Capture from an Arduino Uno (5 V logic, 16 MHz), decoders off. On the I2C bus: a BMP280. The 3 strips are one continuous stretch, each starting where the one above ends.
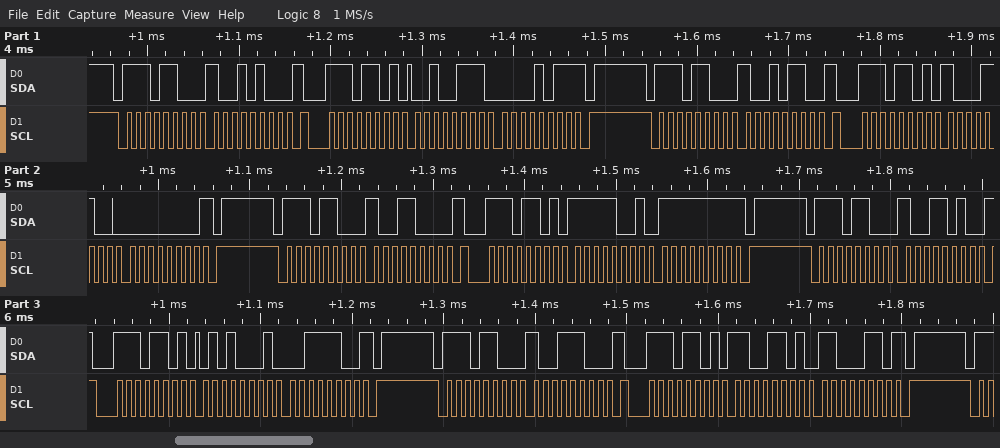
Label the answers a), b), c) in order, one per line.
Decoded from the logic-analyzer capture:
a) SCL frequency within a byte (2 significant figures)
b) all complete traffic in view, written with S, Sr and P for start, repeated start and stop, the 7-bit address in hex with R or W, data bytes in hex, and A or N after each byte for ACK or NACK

a) 100 kHz
b) S 76W A 94 A Sr 76R A 27 A 0B N P S 76W A 96 A Sr 76R A 8C A 00 N P S 76W A 98 A Sr 76R A F9 A FF N P S 76W A 9A A Sr 76R A 51 A 3C N P S 76W A 9C A Sr 76R A CD A C6 N P
